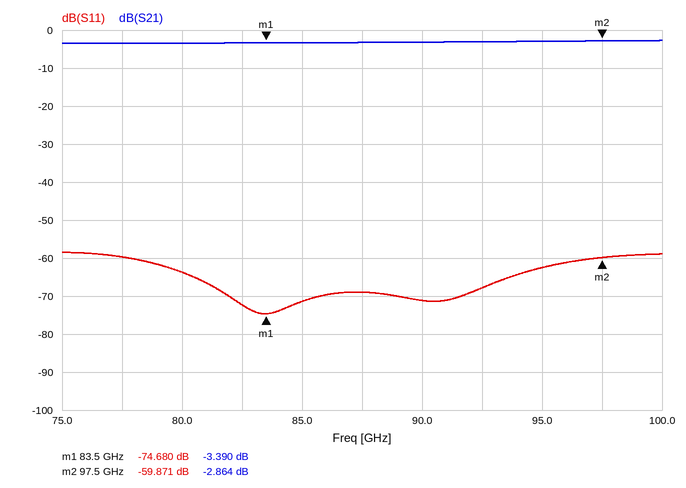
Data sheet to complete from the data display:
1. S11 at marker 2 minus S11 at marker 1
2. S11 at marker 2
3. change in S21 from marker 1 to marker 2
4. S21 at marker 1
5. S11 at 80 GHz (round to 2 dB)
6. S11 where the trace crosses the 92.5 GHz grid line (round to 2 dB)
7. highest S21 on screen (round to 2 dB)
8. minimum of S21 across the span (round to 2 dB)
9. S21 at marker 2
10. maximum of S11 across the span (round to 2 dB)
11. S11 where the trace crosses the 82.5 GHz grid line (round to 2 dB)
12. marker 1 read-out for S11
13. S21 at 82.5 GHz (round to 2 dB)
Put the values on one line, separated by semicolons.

14.809 dB; -59.871 dB; 0.526 dB; -3.390 dB; -64 dB; -68 dB; -2 dB; -4 dB; -2.864 dB; -58 dB; -72 dB; -74.680 dB; -4 dB
